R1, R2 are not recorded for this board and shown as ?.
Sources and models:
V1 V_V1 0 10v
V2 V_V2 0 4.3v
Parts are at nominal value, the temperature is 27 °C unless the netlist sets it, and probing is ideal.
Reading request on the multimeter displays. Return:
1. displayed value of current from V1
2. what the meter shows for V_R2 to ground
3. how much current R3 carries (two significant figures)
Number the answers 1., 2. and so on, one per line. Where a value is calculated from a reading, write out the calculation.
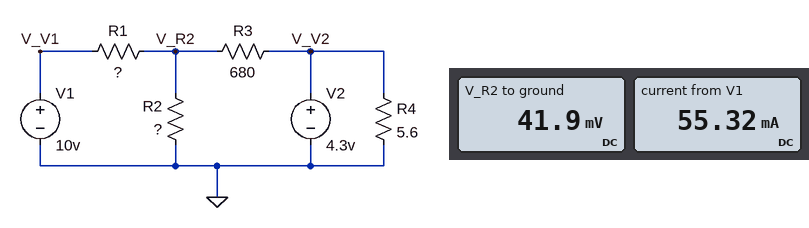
1. 55.32 mA
2. 41.9 mV
3. (4.3 V - 41.9 mV) / 680 Ω = 6.3 mA
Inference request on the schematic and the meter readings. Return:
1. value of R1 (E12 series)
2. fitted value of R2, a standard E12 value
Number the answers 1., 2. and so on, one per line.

1. 180 Ω
2. 0.68 Ω
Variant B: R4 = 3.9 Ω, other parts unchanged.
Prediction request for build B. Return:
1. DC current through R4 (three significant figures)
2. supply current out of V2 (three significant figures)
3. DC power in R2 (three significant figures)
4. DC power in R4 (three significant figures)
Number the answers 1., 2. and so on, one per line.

1. 1.10 A
2. 1.11 A
3. 2.58 mW
4. 4.74 W
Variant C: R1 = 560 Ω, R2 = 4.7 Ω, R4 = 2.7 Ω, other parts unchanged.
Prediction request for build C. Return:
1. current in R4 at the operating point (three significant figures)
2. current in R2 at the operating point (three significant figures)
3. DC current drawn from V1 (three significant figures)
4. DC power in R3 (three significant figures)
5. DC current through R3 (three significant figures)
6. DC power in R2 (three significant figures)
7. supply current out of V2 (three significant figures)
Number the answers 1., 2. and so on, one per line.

1. 1.59 A
2. 23.8 mA
3. 17.7 mA
4. 25.8 mW
5. 6.16 mA
6. 2.67 mW
7. 1.60 A
